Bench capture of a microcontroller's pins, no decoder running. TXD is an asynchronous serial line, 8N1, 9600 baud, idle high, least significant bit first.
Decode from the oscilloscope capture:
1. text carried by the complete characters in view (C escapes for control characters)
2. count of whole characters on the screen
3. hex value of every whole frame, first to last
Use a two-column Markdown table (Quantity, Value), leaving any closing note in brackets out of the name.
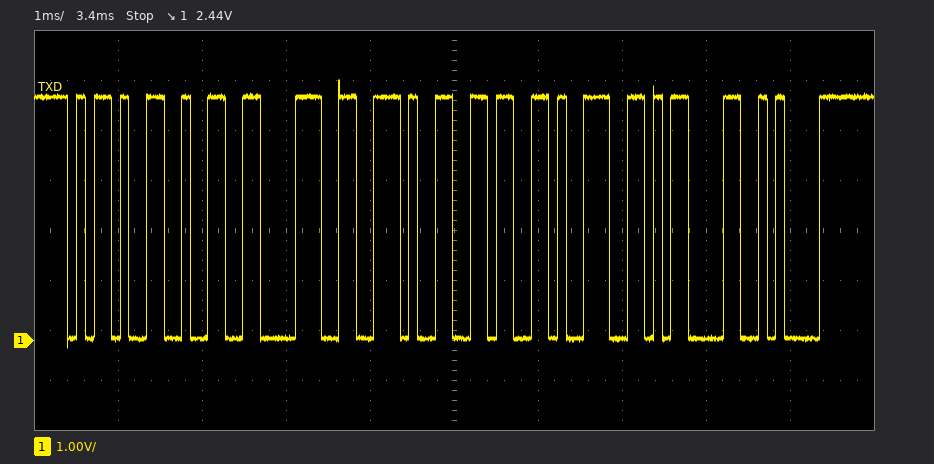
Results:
| Quantity | Value |
|---|---|
| text carried by the complete characters in view | "-28.69\r\n" |
| count of whole characters on the screen | 8 |
| hex value of every whole frame, first to last | 0x2D 0x32 0x38 0x2E 0x36 0x39 0x0D 0x0A |
